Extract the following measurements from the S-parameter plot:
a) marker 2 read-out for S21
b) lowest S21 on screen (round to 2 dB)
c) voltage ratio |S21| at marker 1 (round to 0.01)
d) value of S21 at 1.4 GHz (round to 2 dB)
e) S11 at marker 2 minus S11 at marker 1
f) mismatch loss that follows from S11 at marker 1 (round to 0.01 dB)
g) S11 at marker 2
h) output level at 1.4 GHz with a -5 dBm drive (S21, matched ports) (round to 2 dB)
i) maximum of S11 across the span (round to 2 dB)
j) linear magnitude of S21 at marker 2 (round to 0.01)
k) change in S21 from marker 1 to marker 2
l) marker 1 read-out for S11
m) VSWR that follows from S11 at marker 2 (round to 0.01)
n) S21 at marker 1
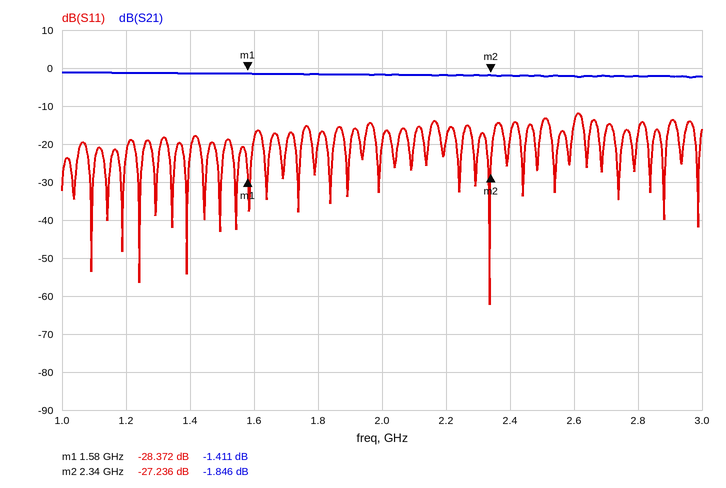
-1.846 dB
-2 dB
0.85
-2 dB
1.136 dB
0.01 dB
-27.236 dB
-6 dBm
-12 dB
0.81
-0.435 dB
-28.372 dB
1.09
-1.411 dB
